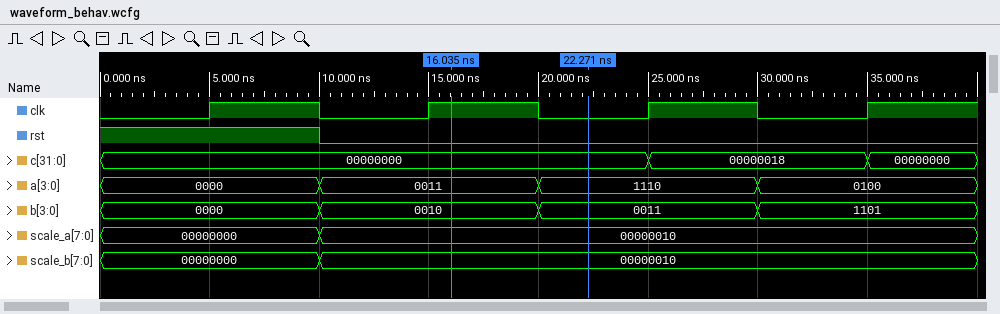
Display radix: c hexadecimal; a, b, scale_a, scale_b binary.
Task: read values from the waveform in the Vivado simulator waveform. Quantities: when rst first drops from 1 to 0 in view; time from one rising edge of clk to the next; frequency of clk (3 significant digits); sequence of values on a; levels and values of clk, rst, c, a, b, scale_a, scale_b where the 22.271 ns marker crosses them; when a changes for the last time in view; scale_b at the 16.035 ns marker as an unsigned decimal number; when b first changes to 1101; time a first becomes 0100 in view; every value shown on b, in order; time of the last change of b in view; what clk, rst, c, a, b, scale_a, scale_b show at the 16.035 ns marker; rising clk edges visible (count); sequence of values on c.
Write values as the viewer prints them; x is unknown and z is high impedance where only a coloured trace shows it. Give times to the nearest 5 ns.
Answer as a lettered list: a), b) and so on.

a) 10 ns
b) 10 ns
c) 100 MHz
d) 0000, 0011, 1110, 0100
e) clk=0, rst=0, c=00000000, a=1110, b=0011, scale_a=00000010, scale_b=00000010
f) 30 ns
g) 2
h) 30 ns
i) 30 ns
j) 0000, 0010, 0011, 1101
k) 30 ns
l) clk=1, rst=0, c=00000000, a=0011, b=0010, scale_a=00000010, scale_b=00000010
m) 4
n) 00000000, 00000018, 00000000
